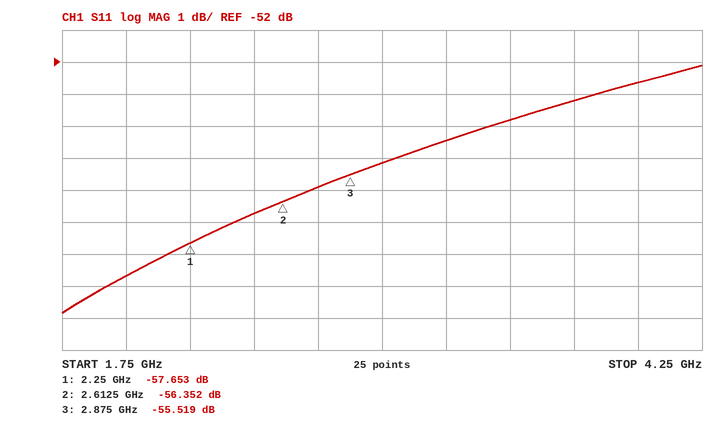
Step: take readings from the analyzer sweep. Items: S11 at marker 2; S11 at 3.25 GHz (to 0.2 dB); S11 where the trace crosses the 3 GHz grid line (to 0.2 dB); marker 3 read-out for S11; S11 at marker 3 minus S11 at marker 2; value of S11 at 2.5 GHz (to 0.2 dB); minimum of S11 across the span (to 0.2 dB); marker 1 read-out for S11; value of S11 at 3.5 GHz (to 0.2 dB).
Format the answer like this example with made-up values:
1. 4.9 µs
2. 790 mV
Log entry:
1. -56.352 dB
2. -54.4 dB
3. -55.2 dB
4. -55.519 dB
5. 0.833 dB
6. -56.8 dB
7. -59.8 dB
8. -57.653 dB
9. -53.8 dB
